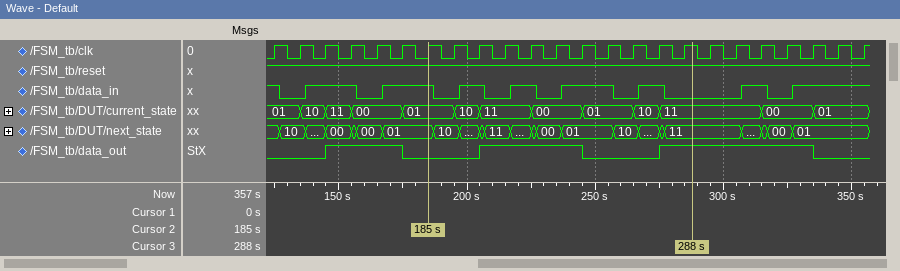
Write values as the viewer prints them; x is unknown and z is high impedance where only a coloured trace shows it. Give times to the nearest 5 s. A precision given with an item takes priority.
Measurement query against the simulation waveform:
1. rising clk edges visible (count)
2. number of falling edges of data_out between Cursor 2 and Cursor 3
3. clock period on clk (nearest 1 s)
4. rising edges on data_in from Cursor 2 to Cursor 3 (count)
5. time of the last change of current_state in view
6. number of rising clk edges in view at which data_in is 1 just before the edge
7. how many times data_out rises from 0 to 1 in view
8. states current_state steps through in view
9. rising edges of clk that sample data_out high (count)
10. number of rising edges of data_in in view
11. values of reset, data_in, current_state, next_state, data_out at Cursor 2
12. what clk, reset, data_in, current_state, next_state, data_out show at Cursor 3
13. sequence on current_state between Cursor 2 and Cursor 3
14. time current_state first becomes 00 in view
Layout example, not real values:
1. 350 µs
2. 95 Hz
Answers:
1. 24
2. 1
3. 10 s
4. 4
5. 335 s
6. 14
7. 3
8. 01, 10, 11, 00, 01, 10, 11, 00, 01, 10, 11, 00, 01
9. 13
10. 8
11. reset=1, data_in=1, current_state=01, next_state=01, data_out=0
12. clk=1, reset=1, data_in=0, current_state=11, next_state=11, data_out=1
13. 01, 10, 11, 00, 01, 10, 11
14. 155 s
